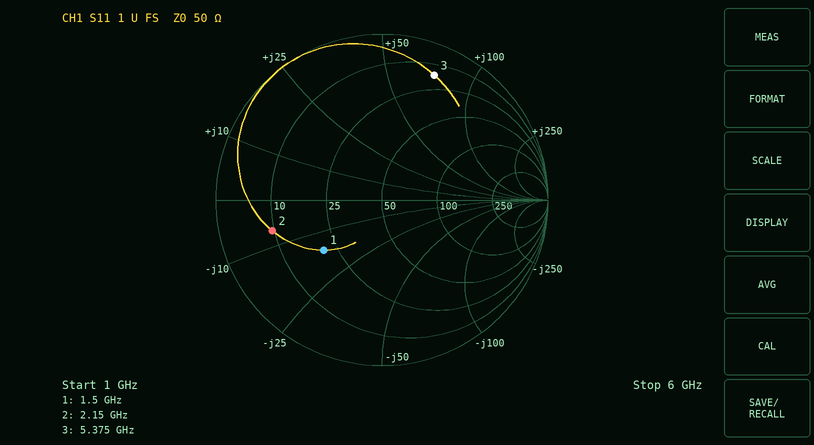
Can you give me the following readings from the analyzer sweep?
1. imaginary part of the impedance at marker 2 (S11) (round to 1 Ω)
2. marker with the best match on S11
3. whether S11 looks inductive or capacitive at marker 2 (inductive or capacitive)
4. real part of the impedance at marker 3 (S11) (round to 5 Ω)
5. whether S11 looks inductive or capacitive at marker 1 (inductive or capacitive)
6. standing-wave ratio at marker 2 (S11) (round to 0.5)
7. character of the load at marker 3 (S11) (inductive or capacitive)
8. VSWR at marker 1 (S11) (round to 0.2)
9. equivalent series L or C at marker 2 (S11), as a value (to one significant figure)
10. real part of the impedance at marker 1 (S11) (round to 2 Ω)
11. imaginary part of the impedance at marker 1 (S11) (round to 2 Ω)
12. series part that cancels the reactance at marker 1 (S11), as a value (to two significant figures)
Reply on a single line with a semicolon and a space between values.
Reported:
-7 Ω; marker 1; capacitive; 15 Ω; capacitive; 5.5; inductive; 2.8; 10 pF; 20 Ω; -16 Ω; 1.7 nH
